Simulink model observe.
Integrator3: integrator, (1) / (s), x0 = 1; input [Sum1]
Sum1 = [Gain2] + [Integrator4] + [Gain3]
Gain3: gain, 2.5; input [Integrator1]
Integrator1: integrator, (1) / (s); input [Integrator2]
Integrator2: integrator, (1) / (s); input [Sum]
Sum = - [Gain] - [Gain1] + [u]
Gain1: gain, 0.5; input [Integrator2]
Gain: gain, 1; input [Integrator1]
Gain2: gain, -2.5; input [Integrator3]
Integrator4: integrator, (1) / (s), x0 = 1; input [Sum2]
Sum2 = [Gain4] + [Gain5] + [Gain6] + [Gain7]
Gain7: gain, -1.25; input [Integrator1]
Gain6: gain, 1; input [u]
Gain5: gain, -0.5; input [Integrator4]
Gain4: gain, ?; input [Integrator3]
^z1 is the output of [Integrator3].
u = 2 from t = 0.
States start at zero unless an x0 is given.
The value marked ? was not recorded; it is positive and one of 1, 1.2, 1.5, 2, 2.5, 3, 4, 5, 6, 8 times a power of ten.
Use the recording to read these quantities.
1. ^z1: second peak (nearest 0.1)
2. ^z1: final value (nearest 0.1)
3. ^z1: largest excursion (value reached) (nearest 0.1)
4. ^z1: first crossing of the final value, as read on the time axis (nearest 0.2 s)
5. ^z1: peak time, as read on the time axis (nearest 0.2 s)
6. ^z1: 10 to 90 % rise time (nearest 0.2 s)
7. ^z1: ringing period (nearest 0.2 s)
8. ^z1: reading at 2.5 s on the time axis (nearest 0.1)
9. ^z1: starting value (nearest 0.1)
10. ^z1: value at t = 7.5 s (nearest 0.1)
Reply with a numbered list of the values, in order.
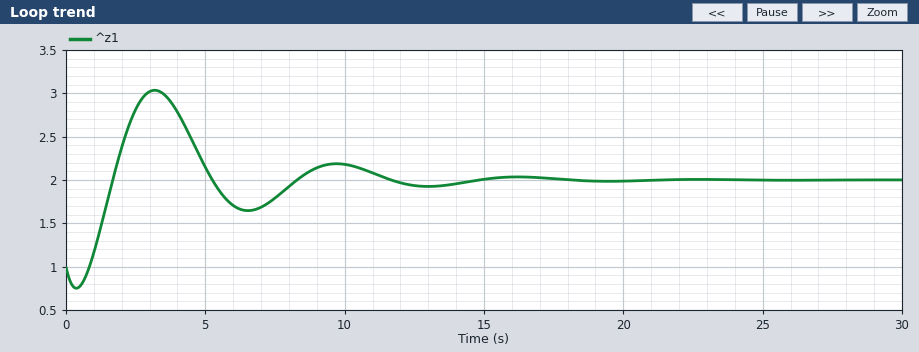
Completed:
1. 2.2
2. 2.0
3. 3.0
4. 1.6 s
5. 3.2 s
6. 0.6 s
7. 6.6 s
8. 2.8
9. 1.0
10. 1.8
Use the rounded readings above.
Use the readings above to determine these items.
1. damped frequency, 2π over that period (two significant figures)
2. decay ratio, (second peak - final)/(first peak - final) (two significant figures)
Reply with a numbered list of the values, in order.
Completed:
1. 0.95 rad/s
2. 0.20
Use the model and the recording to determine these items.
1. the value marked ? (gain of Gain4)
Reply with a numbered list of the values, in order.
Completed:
1. 0.25
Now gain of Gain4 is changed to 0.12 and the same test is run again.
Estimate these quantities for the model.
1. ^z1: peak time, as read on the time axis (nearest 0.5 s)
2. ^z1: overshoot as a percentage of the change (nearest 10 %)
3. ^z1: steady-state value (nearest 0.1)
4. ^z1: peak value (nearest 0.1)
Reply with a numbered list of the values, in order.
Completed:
1. 3.0 s
2. 140 %
3. 1.8
4. 2.9
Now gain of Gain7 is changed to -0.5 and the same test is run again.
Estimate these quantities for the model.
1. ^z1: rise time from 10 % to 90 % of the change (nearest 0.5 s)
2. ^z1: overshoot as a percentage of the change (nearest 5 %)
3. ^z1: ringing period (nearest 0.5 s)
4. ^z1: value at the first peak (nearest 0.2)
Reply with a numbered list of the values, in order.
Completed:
1. 1.5 s
2. 20 %
3. 6.5 s
4. 4.0
